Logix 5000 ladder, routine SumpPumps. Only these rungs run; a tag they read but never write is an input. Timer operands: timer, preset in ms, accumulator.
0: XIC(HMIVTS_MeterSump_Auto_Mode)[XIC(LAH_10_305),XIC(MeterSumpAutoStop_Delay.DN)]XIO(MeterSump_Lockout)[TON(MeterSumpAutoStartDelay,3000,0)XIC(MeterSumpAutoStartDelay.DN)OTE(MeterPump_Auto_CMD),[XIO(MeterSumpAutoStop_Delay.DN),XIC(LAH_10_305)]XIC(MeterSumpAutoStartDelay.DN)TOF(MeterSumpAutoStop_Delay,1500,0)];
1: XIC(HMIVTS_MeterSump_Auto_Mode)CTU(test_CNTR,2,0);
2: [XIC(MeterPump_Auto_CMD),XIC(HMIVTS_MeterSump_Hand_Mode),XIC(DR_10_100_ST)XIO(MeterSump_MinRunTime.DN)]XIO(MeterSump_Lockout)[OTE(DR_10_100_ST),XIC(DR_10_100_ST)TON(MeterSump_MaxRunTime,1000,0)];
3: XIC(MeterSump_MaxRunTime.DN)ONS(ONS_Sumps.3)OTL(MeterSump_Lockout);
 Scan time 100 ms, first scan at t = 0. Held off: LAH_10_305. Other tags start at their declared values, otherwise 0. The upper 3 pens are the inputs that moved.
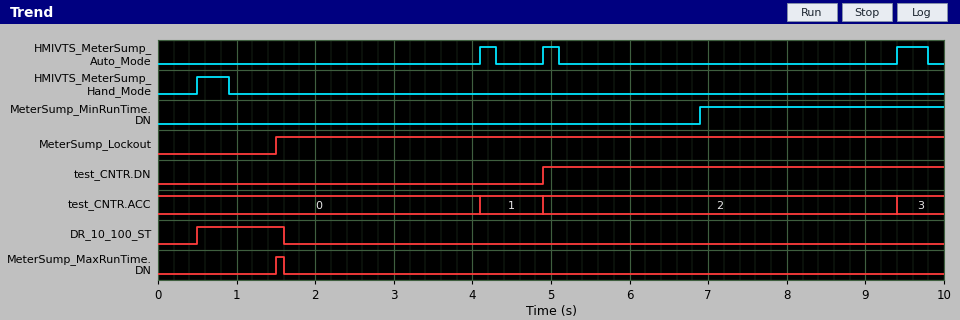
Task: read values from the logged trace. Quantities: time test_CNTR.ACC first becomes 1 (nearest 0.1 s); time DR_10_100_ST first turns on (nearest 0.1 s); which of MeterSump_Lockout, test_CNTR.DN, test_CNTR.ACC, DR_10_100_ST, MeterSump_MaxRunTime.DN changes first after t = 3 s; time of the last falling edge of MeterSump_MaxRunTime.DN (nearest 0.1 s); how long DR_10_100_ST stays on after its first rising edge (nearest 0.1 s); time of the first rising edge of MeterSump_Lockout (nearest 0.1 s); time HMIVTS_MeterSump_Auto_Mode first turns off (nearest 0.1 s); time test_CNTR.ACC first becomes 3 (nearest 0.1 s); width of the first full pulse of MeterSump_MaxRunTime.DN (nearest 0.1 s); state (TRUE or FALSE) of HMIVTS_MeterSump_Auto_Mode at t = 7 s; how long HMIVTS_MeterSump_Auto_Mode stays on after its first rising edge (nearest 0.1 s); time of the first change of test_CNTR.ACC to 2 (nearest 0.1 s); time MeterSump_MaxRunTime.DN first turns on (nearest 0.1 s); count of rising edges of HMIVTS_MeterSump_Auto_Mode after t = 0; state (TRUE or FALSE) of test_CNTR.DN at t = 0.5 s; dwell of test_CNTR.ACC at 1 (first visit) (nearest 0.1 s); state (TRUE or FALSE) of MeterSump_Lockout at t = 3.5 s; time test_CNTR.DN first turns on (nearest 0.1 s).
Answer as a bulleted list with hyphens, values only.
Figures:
- 4.1 s
- 0.5 s
- test_CNTR.ACC
- 1.6 s
- 1.1 s
- 1.5 s
- 4.3 s
- 9.4 s
- 0.1 s
- FALSE
- 0.2 s
- 4.9 s
- 1.5 s
- 3
- FALSE
- 0.8 s
- TRUE
- 4.9 s
